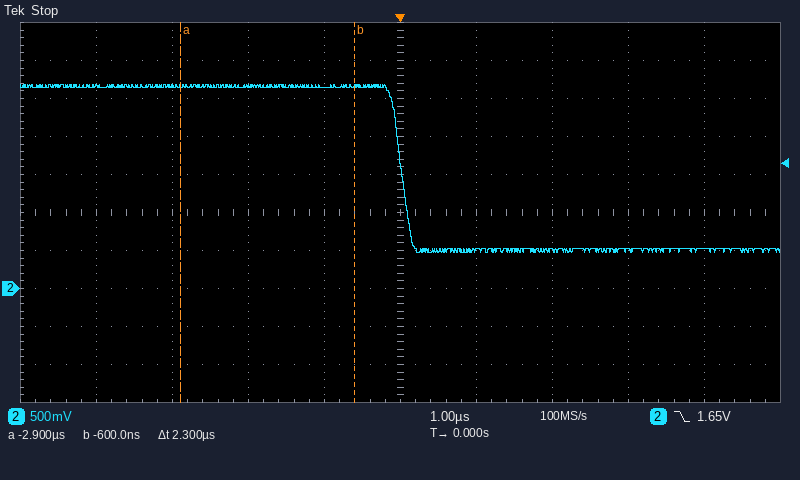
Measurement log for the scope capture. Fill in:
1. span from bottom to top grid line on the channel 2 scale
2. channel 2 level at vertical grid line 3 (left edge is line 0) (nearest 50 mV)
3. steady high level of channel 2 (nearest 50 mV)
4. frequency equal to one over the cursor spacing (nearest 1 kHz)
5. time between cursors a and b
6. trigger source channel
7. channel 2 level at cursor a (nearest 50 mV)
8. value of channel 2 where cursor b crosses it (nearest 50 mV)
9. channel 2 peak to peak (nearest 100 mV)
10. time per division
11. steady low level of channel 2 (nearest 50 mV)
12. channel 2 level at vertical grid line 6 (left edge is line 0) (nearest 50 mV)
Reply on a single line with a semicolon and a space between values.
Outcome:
5 V; 2.65 V; 2.65 V; 435 kHz; 2.3 µs; channel 2; 2.65 V; 2.65 V; 2.20 V; 1 µs; 500 mV; 500 mV
